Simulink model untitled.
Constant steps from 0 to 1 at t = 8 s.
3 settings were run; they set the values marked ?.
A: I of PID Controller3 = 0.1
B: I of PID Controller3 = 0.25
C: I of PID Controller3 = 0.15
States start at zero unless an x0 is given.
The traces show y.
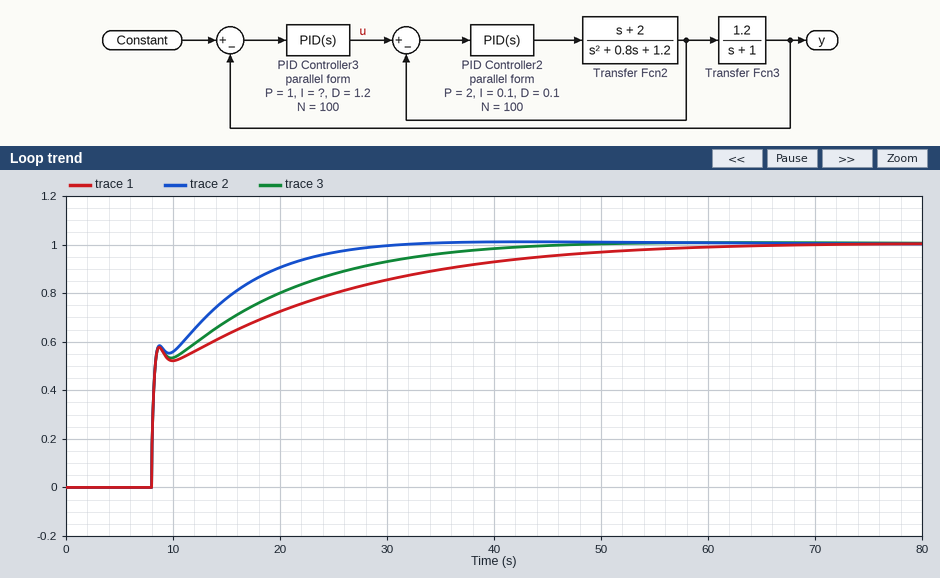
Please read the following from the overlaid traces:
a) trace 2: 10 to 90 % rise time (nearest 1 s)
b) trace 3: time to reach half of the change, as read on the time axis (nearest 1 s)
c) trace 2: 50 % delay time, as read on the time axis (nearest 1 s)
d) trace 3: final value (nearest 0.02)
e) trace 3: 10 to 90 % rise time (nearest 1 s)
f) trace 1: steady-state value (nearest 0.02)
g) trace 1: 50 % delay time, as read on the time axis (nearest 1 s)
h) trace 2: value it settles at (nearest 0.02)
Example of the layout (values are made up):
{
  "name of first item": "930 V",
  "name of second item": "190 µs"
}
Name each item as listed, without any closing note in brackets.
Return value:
{
  "trace 2: 10 to 90 % rise time": "12 s",
  "trace 3: time to reach half of the change, as read on the time axis": "8 s",
  "trace 2: 50 % delay time, as read on the time axis": "8 s",
  "trace 3: final value": "1.00",
  "trace 3: 10 to 90 % rise time": "19 s",
  "trace 1: steady-state value": "1.00",
  "trace 1: 50 % delay time, as read on the time axis": "8 s",
  "trace 2: value it settles at": "1.00"
}
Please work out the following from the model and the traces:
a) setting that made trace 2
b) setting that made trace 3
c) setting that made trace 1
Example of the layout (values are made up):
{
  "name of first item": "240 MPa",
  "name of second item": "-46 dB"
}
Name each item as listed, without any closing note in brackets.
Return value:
{
  "setting that made trace 2": "B",
  "setting that made trace 3": "C",
  "setting that made trace 1": "A"
}
